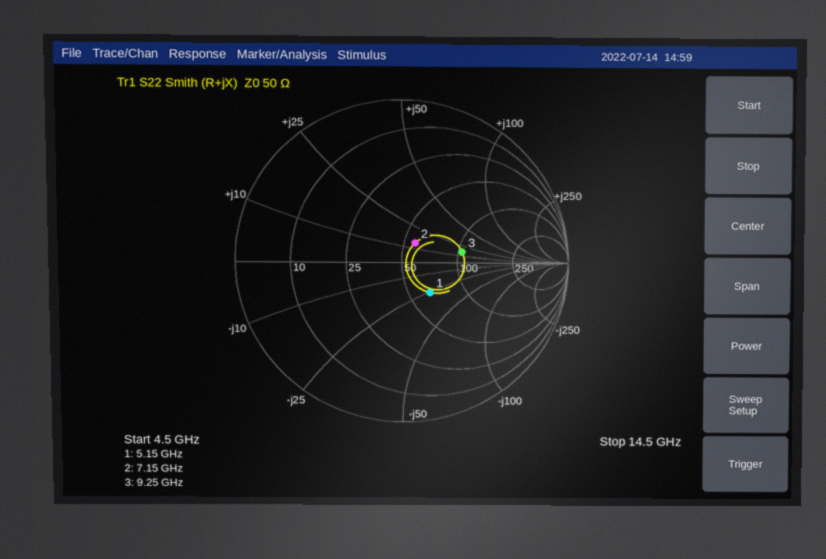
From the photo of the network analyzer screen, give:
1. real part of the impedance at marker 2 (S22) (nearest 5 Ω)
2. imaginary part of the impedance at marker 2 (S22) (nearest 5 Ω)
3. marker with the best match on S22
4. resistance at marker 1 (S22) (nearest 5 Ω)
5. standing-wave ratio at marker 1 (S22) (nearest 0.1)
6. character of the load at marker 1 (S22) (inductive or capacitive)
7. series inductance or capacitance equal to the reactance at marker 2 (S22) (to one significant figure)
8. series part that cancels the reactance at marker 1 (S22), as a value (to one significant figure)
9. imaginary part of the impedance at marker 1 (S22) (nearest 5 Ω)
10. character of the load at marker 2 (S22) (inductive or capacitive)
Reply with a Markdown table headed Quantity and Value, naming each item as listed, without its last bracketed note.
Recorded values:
| Quantity | Value |
|---|---|
| real part of the impedance at marker 2 (S22) | 55 Ω |
| imaginary part of the impedance at marker 2 (S22) | +15 Ω |
| marker with the best match on S22 | marker 2 |
| resistance at marker 1 (S22) | 65 Ω |
| standing-wave ratio at marker 1 (S22) | 1.7 |
| character of the load at marker 1 (S22) | capacitive |
| series inductance or capacitance equal to the reactance at marker 2 (S22) | 300 pH |
| series part that cancels the reactance at marker 1 (S22), as a value | 800 pH |
| imaginary part of the impedance at marker 1 (S22) | -25 Ω |
| character of the load at marker 2 (S22) | inductive |
